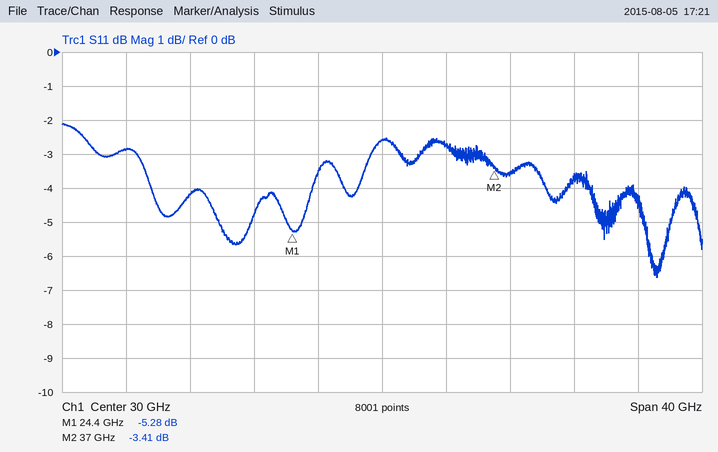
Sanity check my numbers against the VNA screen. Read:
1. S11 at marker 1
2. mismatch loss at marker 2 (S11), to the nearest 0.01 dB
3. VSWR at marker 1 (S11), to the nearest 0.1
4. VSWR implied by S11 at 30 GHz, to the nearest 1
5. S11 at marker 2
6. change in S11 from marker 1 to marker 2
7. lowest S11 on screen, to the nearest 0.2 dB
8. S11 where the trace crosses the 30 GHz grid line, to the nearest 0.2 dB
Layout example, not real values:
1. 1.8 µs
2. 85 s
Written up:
1. -5.28 dB
2. 2.64 dB
3. 3.4
4. 7
5. -3.41 dB
6. 1.87 dB
7. -6.6 dB
8. -2.6 dB
